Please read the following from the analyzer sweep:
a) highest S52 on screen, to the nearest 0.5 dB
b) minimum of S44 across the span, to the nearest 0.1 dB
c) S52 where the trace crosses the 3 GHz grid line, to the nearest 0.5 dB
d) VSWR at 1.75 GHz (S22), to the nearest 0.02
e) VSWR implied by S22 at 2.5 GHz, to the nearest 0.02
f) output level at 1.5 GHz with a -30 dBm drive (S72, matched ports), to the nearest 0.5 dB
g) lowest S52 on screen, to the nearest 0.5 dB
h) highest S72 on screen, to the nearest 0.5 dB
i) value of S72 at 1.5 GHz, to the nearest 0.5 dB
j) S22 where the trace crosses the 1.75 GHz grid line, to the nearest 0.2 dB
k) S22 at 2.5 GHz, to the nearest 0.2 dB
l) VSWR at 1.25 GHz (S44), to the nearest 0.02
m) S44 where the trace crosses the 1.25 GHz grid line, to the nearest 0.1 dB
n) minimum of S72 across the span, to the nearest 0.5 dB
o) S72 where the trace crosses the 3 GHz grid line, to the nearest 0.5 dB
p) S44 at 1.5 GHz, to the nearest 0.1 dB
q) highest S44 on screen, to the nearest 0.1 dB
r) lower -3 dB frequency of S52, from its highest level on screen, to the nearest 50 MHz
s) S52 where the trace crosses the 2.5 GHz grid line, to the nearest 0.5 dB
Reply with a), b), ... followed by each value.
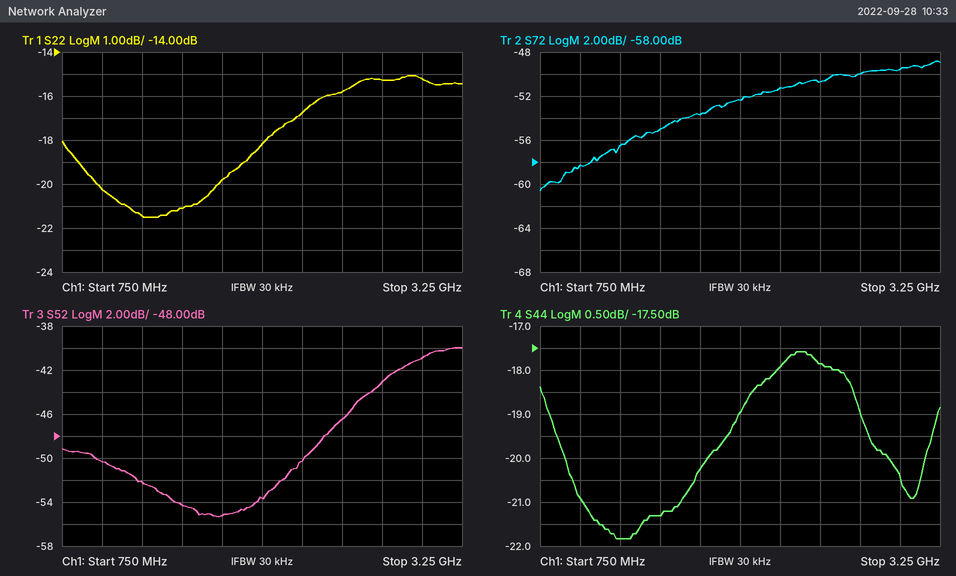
a) -40.0 dB
b) -21.8 dB
c) -41.0 dB
d) 1.22
e) 1.38
f) -85.0 dBm
g) -55.5 dB
h) -49.0 dB
i) -55.0 dB
j) -19.8 dB
k) -15.8 dB
l) 1.18
m) -21.8 dB
n) -60.5 dB
o) -49.5 dB
p) -21.3 dB
q) -17.6 dB
r) 2.75 GHz
s) -46.5 dB
